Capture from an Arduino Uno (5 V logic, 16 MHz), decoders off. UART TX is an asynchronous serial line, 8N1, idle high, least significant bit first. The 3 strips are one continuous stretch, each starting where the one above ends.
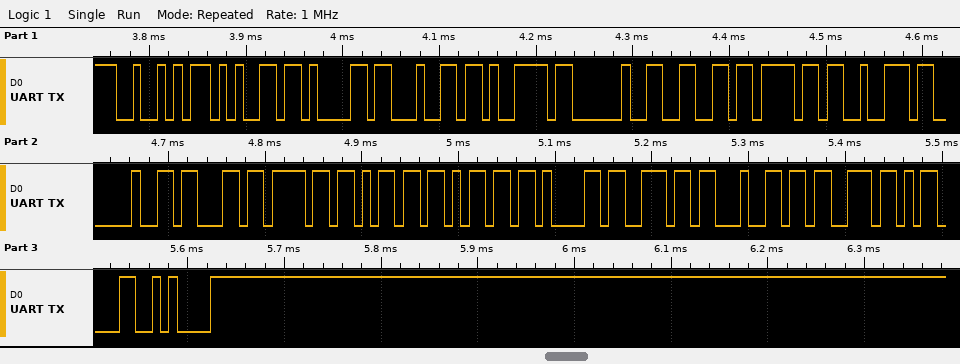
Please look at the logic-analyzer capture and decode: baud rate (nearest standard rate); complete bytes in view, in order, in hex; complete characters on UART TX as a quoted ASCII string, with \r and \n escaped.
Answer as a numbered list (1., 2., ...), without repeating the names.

1. 115200 baud
2. 0x52 0x65 0x61 0x64 0x79 0x20 0x66 0x6F 0x72 0x20 0x63 0x6F 0x6D 0x6D 0x61 0x6E 0x64 0x73 0x0D 0x0A
3. "Ready for commands\r\n"
